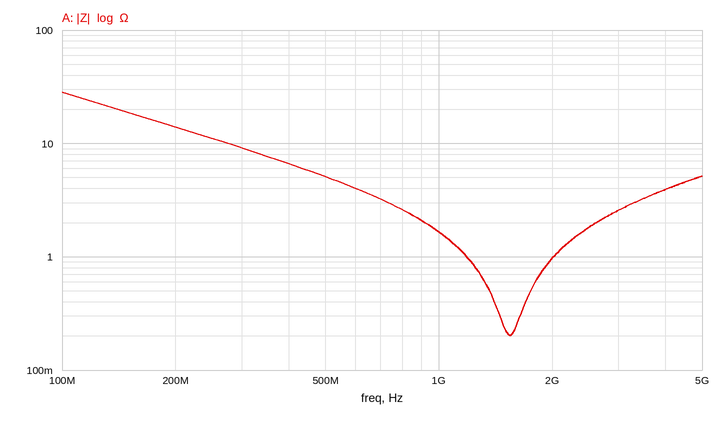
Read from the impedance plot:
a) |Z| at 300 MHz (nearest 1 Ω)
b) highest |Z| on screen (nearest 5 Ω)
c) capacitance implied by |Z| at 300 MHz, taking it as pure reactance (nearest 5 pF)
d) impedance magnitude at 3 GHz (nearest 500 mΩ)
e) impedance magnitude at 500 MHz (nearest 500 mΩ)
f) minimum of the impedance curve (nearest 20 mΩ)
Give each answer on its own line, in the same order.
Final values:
9 Ω
30 Ω
60 pF
2.5 Ω
5.0 Ω
200 mΩ
